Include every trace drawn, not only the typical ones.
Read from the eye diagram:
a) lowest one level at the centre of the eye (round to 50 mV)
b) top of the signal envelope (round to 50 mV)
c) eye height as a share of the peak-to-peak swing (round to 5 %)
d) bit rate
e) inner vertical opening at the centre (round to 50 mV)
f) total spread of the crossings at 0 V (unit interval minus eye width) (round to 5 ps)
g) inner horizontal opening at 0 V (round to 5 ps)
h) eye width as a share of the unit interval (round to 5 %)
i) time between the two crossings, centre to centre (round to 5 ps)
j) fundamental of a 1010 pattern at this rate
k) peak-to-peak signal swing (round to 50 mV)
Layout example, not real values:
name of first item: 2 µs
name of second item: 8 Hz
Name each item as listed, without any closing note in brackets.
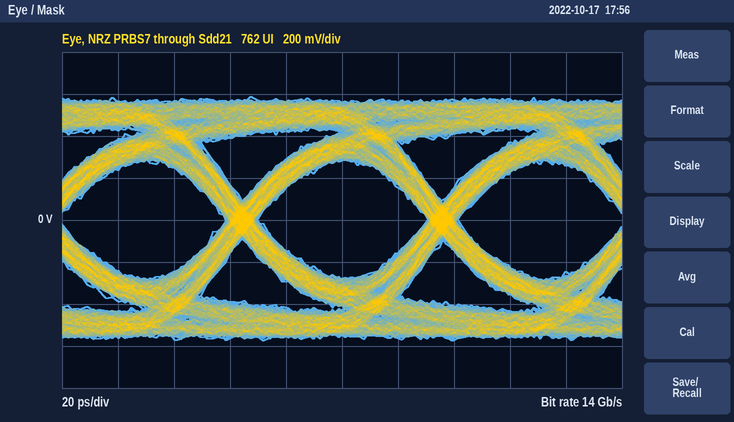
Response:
lowest one level at the centre of the eye: 300 mV
top of the signal envelope: 600 mV
eye height as a share of the peak-to-peak swing: 50 %
bit rate: 14 Gb/s
inner vertical opening at the centre: 550 mV
total spread of the crossings at 0 V (unit interval minus eye width): 10 ps
inner horizontal opening at 0 V: 60 ps
eye width as a share of the unit interval: 85 %
time between the two crossings, centre to centre: 70 ps
fundamental of a 1010 pattern at this rate: 7 GHz
peak-to-peak signal swing: 1.15 V
